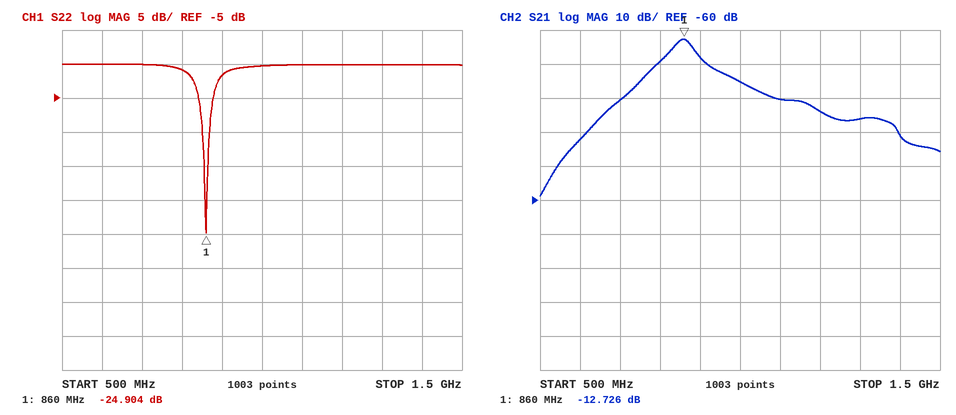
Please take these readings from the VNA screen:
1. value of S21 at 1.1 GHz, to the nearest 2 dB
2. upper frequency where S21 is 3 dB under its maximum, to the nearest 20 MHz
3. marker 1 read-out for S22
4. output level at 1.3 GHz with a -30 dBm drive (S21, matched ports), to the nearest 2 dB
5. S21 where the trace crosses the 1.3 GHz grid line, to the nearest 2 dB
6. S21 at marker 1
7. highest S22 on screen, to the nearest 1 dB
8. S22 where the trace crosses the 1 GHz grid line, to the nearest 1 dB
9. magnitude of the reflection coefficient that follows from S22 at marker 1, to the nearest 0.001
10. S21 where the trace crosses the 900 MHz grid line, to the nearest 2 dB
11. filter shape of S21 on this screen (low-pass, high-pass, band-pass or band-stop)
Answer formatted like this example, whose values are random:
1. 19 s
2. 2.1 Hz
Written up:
1. -30 dB
2. 880 MHz
3. -24.904 dB
4. -66 dBm
5. -36 dB
6. -12.726 dB
7. 0 dB
8. 0 dB
9. 0.057
10. -18 dB
11. band-pass
